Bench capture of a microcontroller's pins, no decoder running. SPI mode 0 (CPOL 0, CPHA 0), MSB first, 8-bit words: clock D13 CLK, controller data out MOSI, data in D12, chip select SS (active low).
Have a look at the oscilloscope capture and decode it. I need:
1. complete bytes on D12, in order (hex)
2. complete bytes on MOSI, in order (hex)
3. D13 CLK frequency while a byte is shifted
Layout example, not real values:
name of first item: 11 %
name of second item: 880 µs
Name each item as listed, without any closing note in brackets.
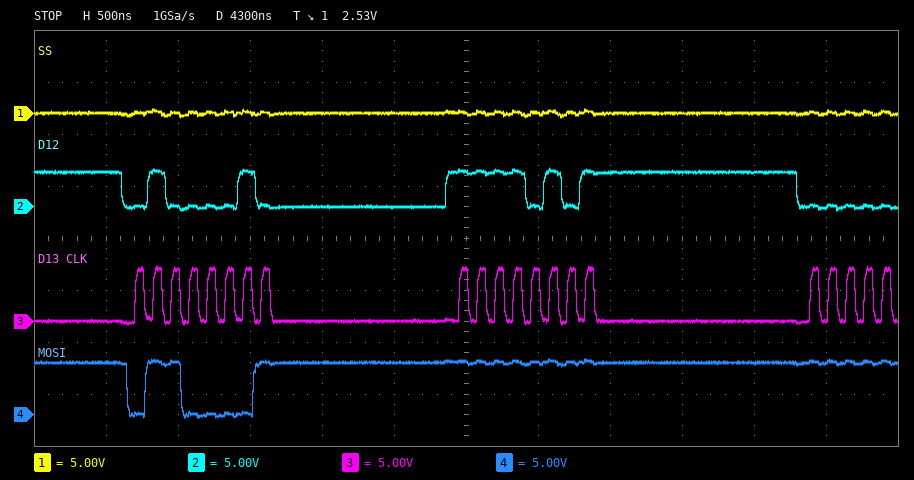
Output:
complete bytes on D12, in order: 42 F5
complete bytes on MOSI, in order: 61 FF
D13 CLK frequency while a byte is shifted: 8 MHz
